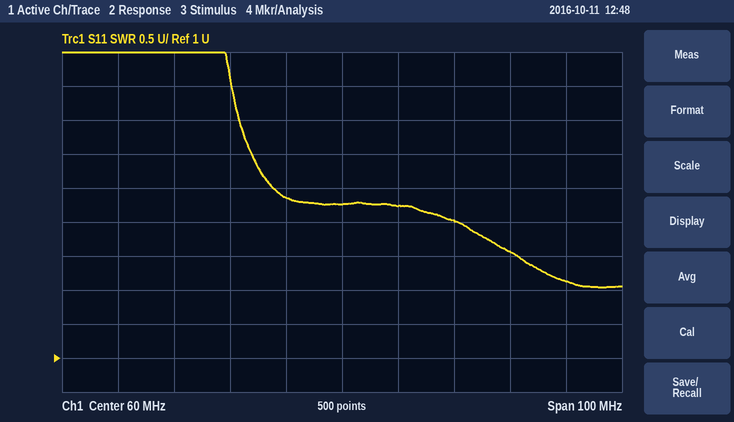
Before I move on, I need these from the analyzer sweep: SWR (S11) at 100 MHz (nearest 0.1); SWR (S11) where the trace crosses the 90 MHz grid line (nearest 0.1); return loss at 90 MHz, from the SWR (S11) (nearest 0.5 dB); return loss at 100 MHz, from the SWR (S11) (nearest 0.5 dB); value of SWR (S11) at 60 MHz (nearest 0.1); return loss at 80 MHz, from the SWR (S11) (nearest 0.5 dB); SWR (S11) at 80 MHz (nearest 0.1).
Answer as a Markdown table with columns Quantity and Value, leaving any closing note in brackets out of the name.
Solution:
| Quantity | Value |
|---|---|
| SWR (S11) at 100 MHz | 2.1 |
| SWR (S11) where the trace crosses the 90 MHz grid line | 2.6 |
| return loss at 90 MHz, from the SWR (S11) | 7.0 dB |
| return loss at 100 MHz, from the SWR (S11) | 9.0 dB |
| value of SWR (S11) at 60 MHz | 3.3 |
| return loss at 80 MHz, from the SWR (S11) | 6.0 dB |
| SWR (S11) at 80 MHz | 3.0 |
